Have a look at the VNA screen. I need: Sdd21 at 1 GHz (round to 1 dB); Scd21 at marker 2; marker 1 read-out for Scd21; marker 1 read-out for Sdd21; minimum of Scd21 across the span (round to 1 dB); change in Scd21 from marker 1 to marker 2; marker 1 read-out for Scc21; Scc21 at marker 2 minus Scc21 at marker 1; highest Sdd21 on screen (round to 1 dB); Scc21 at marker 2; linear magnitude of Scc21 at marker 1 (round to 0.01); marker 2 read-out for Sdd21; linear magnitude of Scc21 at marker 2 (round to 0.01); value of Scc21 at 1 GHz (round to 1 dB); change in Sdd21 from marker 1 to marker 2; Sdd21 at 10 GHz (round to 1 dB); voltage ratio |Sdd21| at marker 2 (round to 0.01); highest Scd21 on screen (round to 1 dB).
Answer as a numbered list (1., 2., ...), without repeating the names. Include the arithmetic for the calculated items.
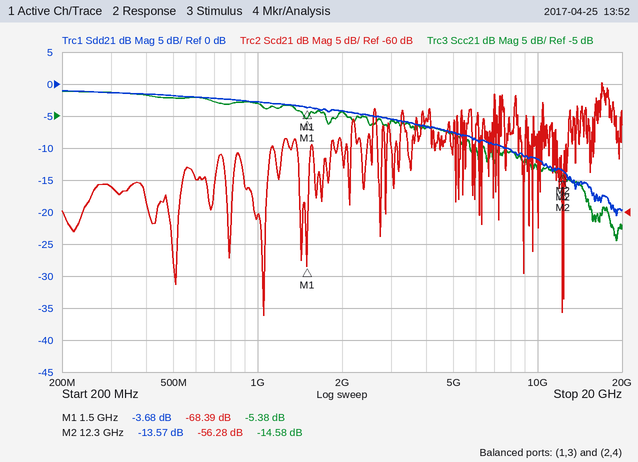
1. -3 dB
2. -56.28 dB
3. -68.39 dB
4. -3.68 dB
5. -76 dB
6. -56.28 − (-68.39) = 12.11 dB
7. -5.38 dB
8. -14.58 − (-5.38) = -9.20 dB
9. -1 dB
10. -14.58 dB
11. 10^(-5.38/20) ≈ 0.54
12. -13.57 dB
13. 10^(-14.58/20) ≈ 0.19
14. -3 dB
15. -13.57 − (-3.68) = -9.89 dB
16. -12 dB
17. 10^(-13.57/20) ≈ 0.21
18. -40 dB
